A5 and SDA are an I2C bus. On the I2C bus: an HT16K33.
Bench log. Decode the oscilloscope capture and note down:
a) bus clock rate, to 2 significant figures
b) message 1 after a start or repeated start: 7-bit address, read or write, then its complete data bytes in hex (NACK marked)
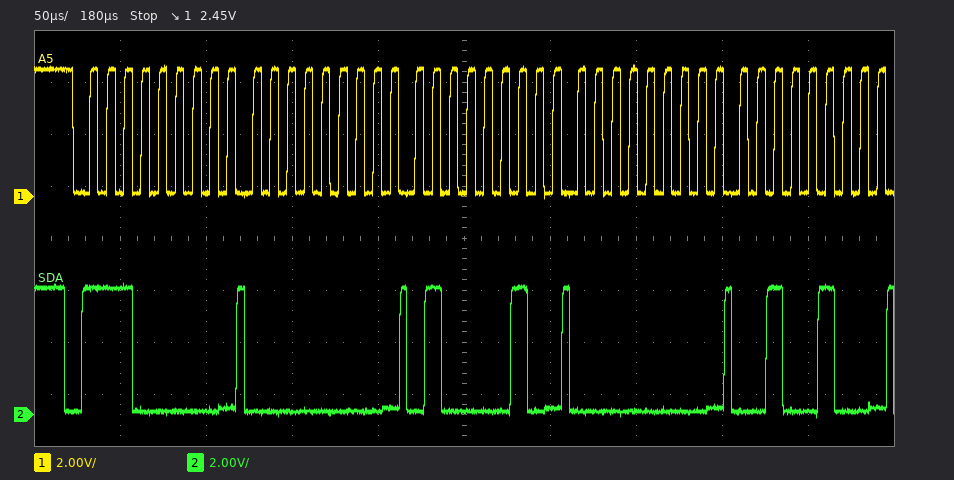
100 kHz
0x70 write: 00 42 00 24
